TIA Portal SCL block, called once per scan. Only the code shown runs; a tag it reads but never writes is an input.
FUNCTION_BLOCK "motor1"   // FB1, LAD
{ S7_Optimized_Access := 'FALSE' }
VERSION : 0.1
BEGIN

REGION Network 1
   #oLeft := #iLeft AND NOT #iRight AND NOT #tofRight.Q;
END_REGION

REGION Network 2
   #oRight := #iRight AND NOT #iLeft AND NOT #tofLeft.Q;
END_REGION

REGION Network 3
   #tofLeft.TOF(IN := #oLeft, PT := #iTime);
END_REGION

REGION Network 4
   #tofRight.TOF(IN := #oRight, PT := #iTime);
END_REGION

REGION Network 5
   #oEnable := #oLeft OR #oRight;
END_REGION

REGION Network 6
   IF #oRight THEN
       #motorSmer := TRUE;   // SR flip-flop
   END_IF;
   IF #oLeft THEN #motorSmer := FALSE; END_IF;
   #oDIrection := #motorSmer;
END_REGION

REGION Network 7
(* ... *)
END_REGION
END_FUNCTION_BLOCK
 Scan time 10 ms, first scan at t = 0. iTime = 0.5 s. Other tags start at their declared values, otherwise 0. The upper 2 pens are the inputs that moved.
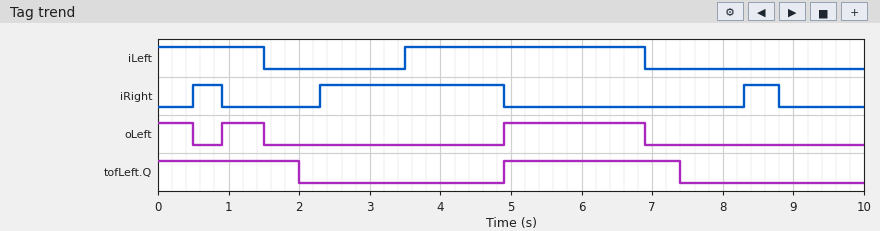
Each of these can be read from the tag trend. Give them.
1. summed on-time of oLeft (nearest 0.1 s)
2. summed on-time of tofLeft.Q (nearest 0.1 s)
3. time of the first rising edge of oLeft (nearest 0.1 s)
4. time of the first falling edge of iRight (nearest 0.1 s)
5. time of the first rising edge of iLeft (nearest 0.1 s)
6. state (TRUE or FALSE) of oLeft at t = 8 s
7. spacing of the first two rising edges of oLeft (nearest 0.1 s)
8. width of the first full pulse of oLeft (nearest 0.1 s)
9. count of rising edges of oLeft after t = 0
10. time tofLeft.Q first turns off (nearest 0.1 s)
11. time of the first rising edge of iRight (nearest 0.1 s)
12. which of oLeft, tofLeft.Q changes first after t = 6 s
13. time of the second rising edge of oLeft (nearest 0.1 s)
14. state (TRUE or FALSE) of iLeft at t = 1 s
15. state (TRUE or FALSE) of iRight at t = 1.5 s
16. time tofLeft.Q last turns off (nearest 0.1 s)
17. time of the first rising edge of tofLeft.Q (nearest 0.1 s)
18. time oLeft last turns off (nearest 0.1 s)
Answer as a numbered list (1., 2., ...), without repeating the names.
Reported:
1. 3.1 s
2. 4.5 s
3. 0.9 s
4. 0.9 s
5. 3.5 s
6. FALSE
7. 4.0 s
8. 0.6 s
9. 2
10. 2.0 s
11. 0.5 s
12. oLeft
13. 4.9 s
14. TRUE
15. FALSE
16. 7.4 s
17. 4.9 s
18. 6.9 s
